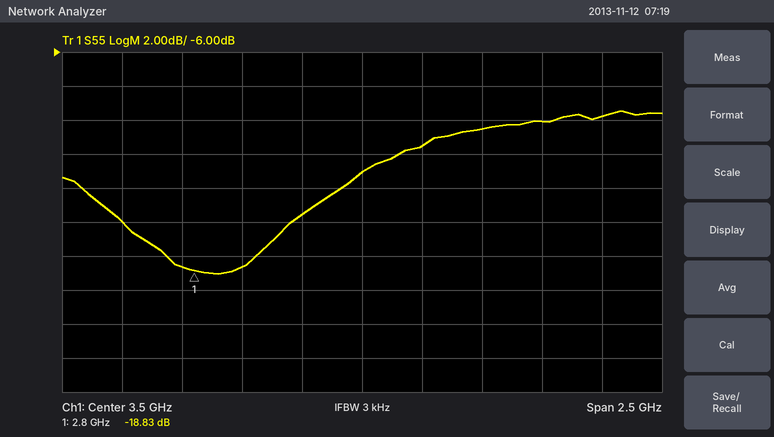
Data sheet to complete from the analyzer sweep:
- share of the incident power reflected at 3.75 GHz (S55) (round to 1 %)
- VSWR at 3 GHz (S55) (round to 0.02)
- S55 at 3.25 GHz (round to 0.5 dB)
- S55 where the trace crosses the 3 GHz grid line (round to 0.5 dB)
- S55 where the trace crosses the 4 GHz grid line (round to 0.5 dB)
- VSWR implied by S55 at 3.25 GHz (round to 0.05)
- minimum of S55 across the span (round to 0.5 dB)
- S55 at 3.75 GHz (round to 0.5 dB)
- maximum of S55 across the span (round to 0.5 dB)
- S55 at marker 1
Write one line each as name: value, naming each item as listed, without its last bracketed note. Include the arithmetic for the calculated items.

share of the incident power reflected at 3.75 GHz (S55): 10^(-11.5/10) ≈ 7 %
VSWR at 3 GHz (S55): |Γ| = 10^(-18.5/20) = 0.1189; VSWR = (1 + 0.1189)/(1 − 0.1189) ≈ 1.27, so 1.26 to the nearest 0.02
S55 at 3.25 GHz: -15.5 dB
S55 where the trace crosses the 3 GHz grid line: -18.5 dB
S55 where the trace crosses the 4 GHz grid line: -10.5 dB
VSWR implied by S55 at 3.25 GHz: |Γ| = 10^(-15.5/20) = 0.1679; VSWR = (1 + 0.1679)/(1 − 0.1679) ≈ 1.40
minimum of S55 across the span: -19.0 dB
S55 at 3.75 GHz: -11.5 dB
maximum of S55 across the span: -9.5 dB
S55 at marker 1: -18.83 dB
